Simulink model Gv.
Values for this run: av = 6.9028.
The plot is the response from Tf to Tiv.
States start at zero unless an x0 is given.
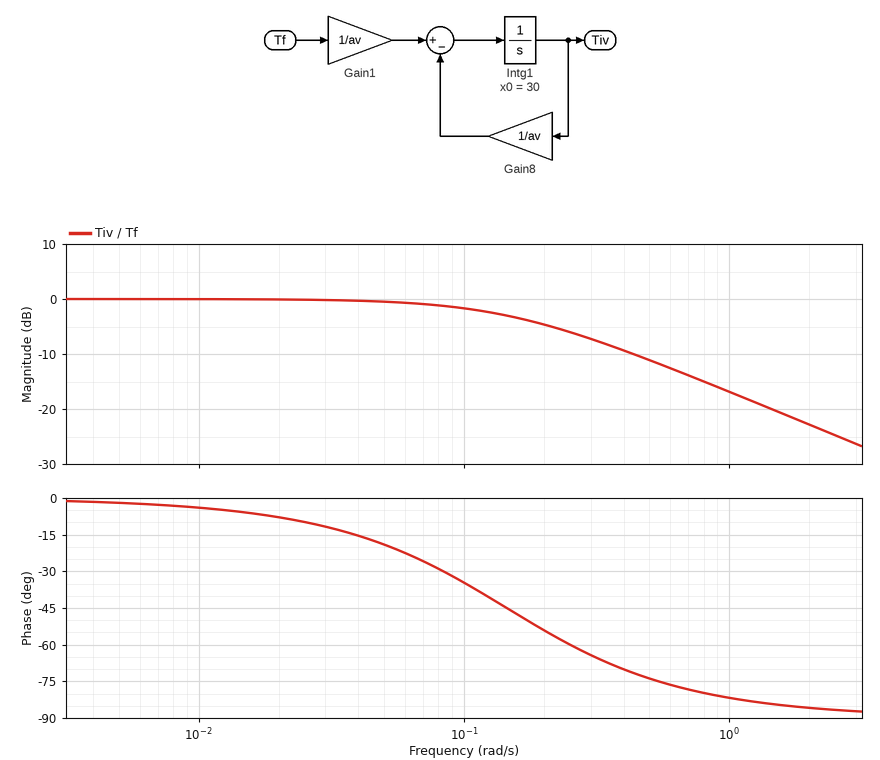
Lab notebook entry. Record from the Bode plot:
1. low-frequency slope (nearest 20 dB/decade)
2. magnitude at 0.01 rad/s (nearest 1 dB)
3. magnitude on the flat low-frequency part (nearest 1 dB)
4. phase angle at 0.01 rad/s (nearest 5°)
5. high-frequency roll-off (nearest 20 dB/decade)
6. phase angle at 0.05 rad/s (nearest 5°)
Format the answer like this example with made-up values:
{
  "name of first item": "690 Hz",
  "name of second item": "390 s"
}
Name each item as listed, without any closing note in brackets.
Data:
{
  "low-frequency slope": "0 dB/decade",
  "magnitude at 0.01 rad/s": "0 dB",
  "magnitude on the flat low-frequency part": "0 dB",
  "phase angle at 0.01 rad/s": "-5°",
  "high-frequency roll-off": "-20 dB/decade",
  "phase angle at 0.05 rad/s": "-20°"
}
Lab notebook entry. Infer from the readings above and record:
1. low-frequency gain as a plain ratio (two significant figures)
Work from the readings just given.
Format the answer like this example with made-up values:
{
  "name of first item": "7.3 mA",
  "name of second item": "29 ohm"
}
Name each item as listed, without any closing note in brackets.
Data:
{
  "low-frequency gain as a plain ratio": "1.0"
}
